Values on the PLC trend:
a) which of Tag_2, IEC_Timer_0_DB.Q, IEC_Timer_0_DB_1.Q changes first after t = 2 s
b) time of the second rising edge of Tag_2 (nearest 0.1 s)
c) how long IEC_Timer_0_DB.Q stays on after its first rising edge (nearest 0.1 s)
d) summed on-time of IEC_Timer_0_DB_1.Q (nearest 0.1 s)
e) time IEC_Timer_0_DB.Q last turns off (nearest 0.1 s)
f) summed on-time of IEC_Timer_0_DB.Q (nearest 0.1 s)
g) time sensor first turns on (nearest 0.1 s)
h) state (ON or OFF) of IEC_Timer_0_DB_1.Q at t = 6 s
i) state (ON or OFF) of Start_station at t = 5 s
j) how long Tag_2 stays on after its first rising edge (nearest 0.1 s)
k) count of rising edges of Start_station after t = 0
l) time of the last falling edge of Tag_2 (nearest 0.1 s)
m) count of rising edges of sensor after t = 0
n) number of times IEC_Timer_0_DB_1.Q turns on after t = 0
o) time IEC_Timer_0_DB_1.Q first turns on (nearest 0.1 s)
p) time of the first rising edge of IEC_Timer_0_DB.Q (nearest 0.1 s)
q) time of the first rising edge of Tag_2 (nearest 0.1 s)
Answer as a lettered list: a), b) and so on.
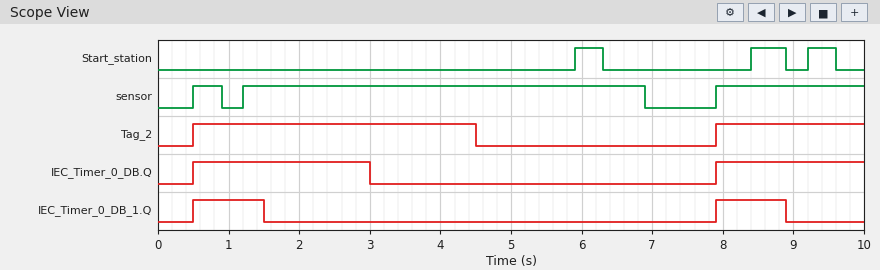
a) IEC_Timer_0_DB.Q
b) 7.9 s
c) 2.5 s
d) 2.0 s
e) 3.0 s
f) 4.6 s
g) 0.5 s
h) OFF
i) OFF
j) 4.0 s
k) 3
l) 4.5 s
m) 3
n) 2
o) 0.5 s
p) 0.5 s
q) 0.5 s
